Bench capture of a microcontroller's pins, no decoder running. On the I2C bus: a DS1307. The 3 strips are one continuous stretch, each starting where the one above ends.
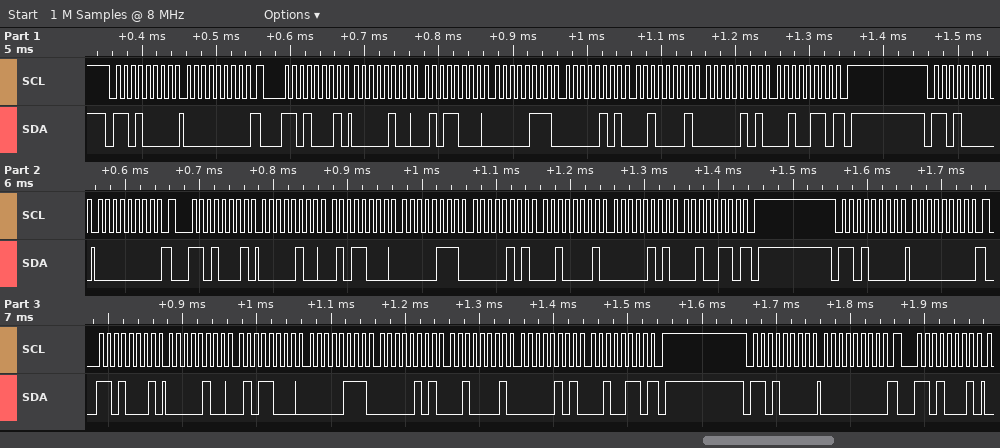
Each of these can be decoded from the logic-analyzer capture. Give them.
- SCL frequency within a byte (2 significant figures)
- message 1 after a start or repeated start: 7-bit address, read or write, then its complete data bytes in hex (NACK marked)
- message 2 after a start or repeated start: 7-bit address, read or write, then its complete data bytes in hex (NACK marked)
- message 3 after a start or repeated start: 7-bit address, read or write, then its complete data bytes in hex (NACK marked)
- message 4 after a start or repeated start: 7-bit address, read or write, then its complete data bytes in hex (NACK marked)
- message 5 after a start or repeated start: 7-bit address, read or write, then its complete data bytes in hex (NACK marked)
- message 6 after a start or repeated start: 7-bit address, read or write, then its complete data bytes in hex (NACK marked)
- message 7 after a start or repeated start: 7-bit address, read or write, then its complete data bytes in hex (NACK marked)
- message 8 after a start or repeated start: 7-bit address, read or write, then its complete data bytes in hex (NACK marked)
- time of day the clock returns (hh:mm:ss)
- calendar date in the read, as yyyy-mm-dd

100 kHz
0x68 write: 00
0x68 read: 04 58 07 05 21 05 26 NACK
0x68 write: 00
0x68 read: 04 58 07 05 21 05 26 NACK
0x68 write: 00
0x68 read: 04 58 07 05 21 05 26 NACK
0x68 write: 00
0x68 read
07:58:04
2026-05-21
